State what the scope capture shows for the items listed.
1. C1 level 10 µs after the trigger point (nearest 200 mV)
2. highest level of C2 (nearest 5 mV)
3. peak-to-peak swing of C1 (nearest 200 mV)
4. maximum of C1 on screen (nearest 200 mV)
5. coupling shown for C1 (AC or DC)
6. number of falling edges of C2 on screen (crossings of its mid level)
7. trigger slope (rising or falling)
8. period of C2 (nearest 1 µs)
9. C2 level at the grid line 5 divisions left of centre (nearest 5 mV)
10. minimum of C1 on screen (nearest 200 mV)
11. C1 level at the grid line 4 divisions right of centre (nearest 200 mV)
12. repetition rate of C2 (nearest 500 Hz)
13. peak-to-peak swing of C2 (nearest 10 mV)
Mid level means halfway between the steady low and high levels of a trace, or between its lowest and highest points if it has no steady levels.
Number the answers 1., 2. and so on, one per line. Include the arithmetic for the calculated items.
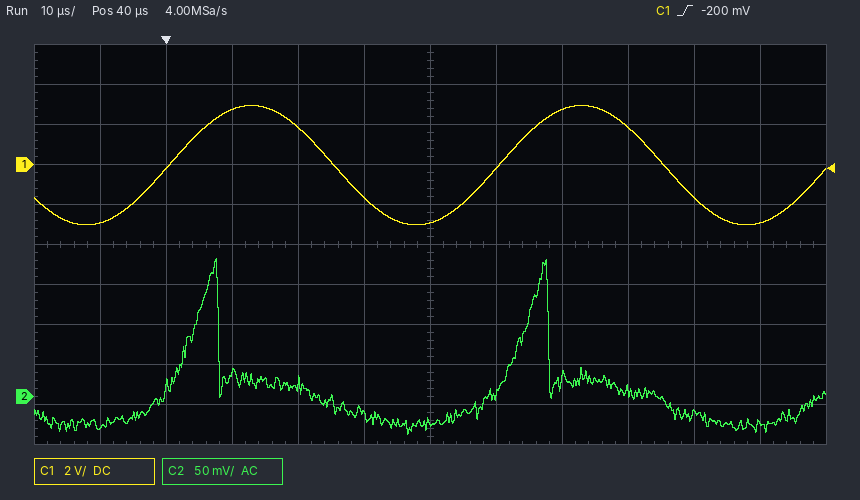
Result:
1. 2.8 V
2. 170 mV
3. 3.0 V − (-3.0 V) = 6.0 V
4. 3.0 V
5. DC
6. 2
7. rising
8. 50 µs
9. -40 mV
10. -3.0 V
11. -1.6 V
12. 1 / 50 µs ≈ 20.0 kHz
13. 220 mV
